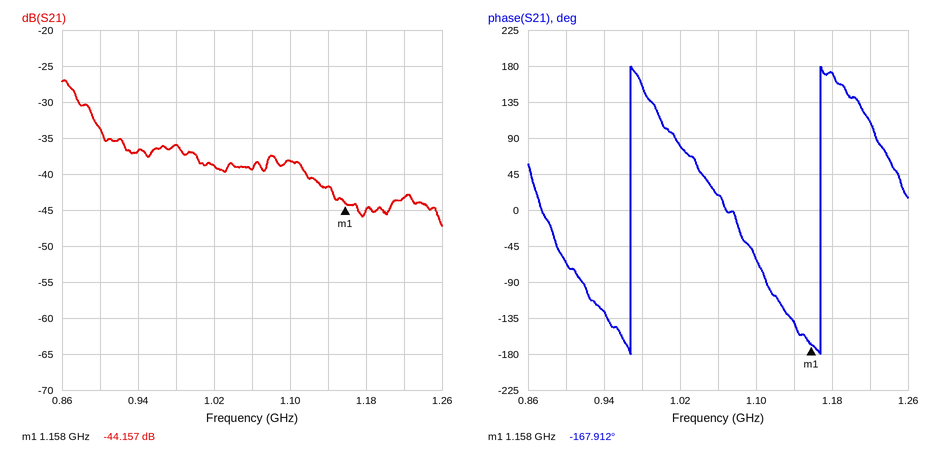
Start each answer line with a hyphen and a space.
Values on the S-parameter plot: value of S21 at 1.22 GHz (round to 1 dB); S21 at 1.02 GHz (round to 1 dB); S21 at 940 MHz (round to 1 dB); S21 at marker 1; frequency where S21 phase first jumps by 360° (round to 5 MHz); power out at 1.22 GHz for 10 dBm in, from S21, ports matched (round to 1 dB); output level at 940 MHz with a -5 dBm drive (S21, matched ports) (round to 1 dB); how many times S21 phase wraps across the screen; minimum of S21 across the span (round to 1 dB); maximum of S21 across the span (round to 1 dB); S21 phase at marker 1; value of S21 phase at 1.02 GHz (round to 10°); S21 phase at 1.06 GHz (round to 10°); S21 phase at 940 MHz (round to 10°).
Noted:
- -43 dB
- -39 dB
- -37 dB
- -44.157 dB
- 970 MHz
- -33 dBm
- -42 dBm
- 2
- -47 dB
- -27 dB
- -167.912°
- 80°
- 20°
- -130°
